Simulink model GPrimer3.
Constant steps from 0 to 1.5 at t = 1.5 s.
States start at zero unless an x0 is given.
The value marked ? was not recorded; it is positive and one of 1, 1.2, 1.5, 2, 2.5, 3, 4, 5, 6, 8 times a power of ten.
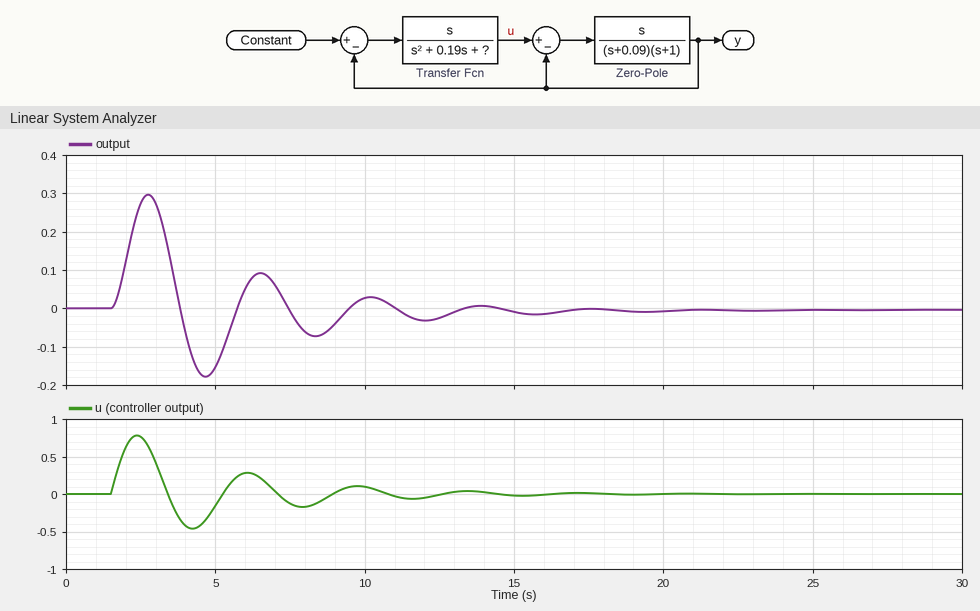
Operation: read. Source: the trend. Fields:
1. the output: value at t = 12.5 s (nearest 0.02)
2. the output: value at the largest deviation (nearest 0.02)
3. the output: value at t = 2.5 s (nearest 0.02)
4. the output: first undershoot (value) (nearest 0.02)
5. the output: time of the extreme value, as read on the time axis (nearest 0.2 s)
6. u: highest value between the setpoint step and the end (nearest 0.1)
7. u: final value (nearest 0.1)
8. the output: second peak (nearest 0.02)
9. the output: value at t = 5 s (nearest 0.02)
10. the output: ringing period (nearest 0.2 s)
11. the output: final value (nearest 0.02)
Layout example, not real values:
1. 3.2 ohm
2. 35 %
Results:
1. -0.02
2. 0.30
3. 0.28
4. -0.18
5. 2.8 s
6. 0.8
7. 0.0
8. 0.10
9. -0.16
10. 3.8 s
11. 0.00
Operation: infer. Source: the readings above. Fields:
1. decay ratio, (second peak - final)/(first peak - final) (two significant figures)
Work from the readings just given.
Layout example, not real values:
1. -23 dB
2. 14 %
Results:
1. 0.33
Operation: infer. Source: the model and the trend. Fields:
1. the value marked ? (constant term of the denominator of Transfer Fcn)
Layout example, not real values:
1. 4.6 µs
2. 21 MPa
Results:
1. 2.5
